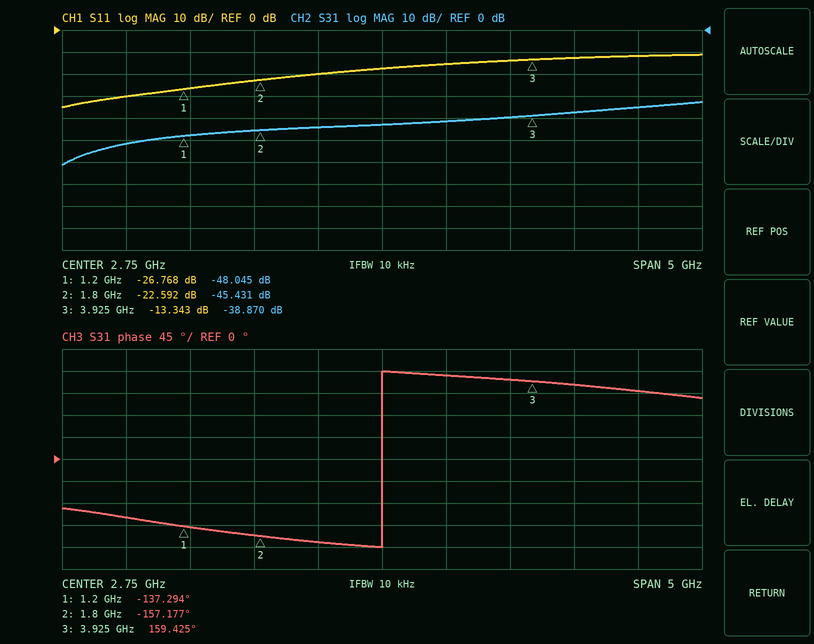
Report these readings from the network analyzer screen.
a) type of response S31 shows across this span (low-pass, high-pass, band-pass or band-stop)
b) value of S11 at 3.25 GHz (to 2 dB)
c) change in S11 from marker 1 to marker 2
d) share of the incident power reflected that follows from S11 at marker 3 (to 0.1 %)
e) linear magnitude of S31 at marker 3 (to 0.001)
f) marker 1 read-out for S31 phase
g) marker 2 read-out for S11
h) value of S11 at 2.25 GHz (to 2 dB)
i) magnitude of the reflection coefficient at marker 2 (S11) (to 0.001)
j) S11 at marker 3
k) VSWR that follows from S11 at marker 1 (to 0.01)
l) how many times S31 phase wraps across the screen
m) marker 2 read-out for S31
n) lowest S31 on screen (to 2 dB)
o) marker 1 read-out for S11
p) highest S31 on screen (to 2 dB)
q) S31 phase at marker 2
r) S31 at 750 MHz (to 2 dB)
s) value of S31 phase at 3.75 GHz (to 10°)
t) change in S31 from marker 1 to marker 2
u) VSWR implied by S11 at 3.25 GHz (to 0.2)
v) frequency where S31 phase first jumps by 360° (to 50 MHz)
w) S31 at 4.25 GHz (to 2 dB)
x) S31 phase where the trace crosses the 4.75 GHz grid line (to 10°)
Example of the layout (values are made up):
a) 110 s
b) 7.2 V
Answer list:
a) high-pass
b) -16 dB
c) 4.176 dB
d) 4.6 %
e) 0.011
f) -137.294°
g) -22.592 dB
h) -20 dB
i) 0.074
j) -13.343 dB
k) 1.10
l) 1
m) -45.431 dB
n) -62 dB
o) -26.768 dB
p) -32 dB
q) -157.177°
r) -52 dB
s) 160°
t) 2.614 dB
u) 1.4
v) 2.75 GHz
w) -38 dB
x) 140°
